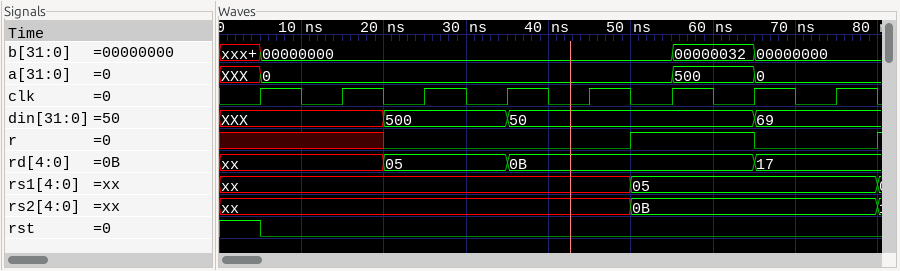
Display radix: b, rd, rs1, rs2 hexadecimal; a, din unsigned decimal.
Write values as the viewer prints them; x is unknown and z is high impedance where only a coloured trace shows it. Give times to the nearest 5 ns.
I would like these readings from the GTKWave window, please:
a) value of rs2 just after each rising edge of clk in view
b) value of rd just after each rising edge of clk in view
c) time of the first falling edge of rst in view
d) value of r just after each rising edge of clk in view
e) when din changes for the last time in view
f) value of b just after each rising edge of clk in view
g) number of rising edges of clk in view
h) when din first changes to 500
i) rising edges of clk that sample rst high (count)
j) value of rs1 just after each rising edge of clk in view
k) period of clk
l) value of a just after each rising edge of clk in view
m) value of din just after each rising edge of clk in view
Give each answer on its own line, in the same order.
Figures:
xx, xx, xx, xx, xx, 0B, 0B, 0B
xx, xx, 05, 0B, 0B, 0B, 17, 17
5 ns
x x 0 0 0 1 0 0
65 ns
00000000, 00000000, 00000000, 00000000, 00000000, 00000032, 00000000, 00000000
8
20 ns
1
xx, xx, xx, xx, xx, 05, 05, 05
10 ns
0, 0, 0, 0, 0, 500, 0, 0
XXX, XXX, 500, 50, 50, 50, 69, 69
